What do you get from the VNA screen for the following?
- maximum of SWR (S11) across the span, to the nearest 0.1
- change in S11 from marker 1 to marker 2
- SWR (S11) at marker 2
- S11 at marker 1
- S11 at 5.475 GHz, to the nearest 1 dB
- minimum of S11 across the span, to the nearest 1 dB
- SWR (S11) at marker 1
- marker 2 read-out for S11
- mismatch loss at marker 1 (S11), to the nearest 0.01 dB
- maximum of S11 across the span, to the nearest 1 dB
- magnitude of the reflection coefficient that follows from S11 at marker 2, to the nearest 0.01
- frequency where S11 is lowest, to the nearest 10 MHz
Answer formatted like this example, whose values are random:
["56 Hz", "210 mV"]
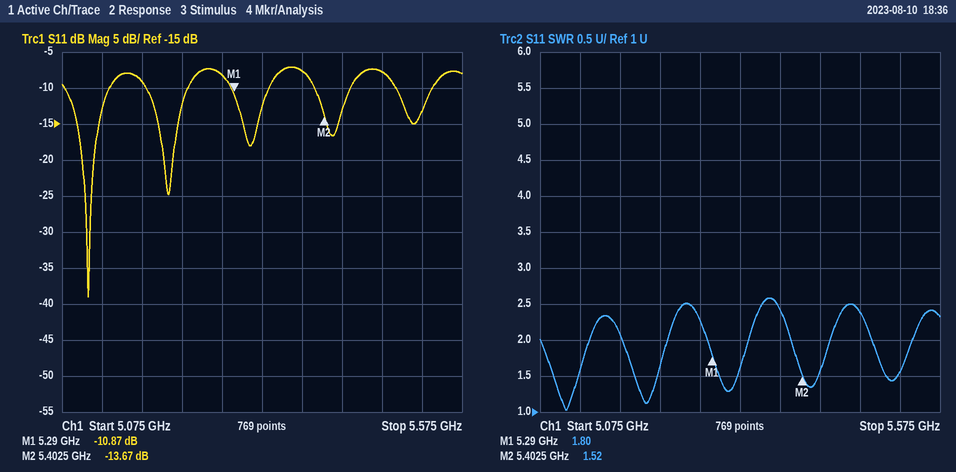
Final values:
["2.6", "-2.80 dB", "1.52", "-10.87 dB", "-8 dB", "-39 dB", "1.80", "-13.67 dB", "0.37 dB", "-7 dB", "0.21", "5.11 GHz"]
